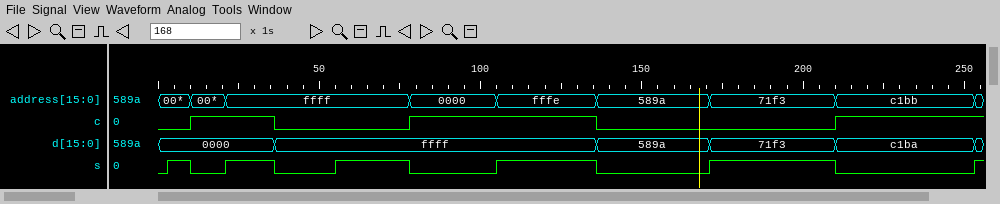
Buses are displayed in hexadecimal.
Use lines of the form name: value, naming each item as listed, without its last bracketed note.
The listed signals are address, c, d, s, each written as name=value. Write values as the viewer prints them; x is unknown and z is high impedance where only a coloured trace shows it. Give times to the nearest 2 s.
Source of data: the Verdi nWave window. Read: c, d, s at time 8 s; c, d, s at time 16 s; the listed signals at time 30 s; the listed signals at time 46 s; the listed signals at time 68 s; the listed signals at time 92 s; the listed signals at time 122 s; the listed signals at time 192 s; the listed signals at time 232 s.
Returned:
c, d, s at time 8 s: c=0, d=0000, s=1
c, d, s at time 16 s: c=1, d=0000, s=0
the listed signals at time 30 s: address=ffff, c=1, d=0000, s=1
the listed signals at time 46 s: address=ffff, c=0, d=ffff, s=0
the listed signals at time 68 s: address=ffff, c=0, d=ffff, s=1
the listed signals at time 92 s: address=0000, c=1, d=ffff, s=0
the listed signals at time 122 s: address=fffe, c=1, d=ffff, s=1
the listed signals at time 192 s: address=71f3, c=0, d=71f3, s=1
the listed signals at time 232 s: address=c1bb, c=1, d=c1ba, s=0
